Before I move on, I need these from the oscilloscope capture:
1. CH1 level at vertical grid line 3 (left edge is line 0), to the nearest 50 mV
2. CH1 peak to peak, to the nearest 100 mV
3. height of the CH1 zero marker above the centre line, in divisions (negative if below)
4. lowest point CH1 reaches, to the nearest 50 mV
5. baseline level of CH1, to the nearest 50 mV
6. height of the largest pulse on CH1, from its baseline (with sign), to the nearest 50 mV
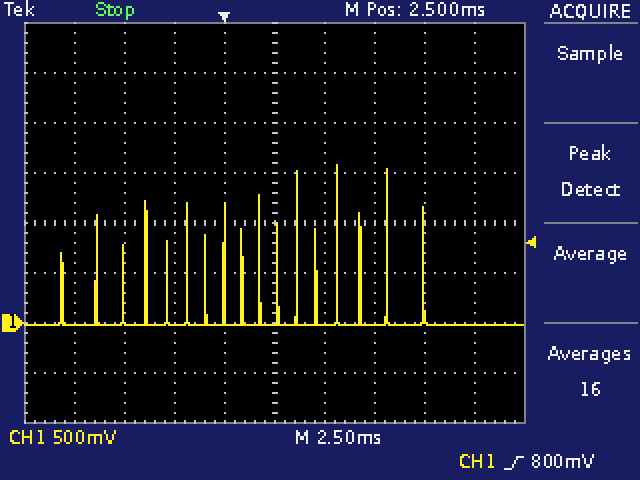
0 mV
1.60 V
-2.0 div
0 mV
0 mV
+1.60 V
